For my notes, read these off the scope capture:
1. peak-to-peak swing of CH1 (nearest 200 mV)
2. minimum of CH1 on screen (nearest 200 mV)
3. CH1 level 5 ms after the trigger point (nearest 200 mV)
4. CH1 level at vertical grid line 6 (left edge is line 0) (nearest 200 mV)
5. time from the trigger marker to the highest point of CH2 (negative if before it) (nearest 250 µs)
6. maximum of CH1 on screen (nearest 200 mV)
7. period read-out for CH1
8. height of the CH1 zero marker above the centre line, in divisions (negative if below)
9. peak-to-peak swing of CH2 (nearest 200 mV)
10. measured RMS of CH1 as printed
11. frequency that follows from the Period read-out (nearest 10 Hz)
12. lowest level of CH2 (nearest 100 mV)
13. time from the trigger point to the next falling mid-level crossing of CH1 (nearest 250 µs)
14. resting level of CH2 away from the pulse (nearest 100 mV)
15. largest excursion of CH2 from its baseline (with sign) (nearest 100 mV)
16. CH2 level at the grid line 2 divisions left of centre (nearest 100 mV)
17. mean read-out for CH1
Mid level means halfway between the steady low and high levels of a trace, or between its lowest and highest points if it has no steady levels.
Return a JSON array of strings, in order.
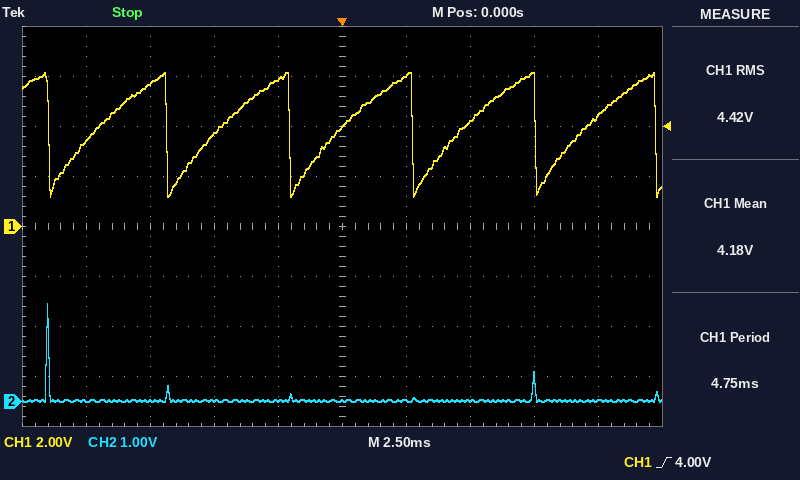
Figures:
["5.0 V", "1.2 V", "4.2 V", "6.0 V", "-11.50 ms", "6.2 V", "4.75 ms", "0.0 div", "2.0 V", "4.42 V", "210 Hz", "0.0 V", "2.75 ms", "0.0 V", "+1.9 V", "0.0 V", "4.18 V"]
